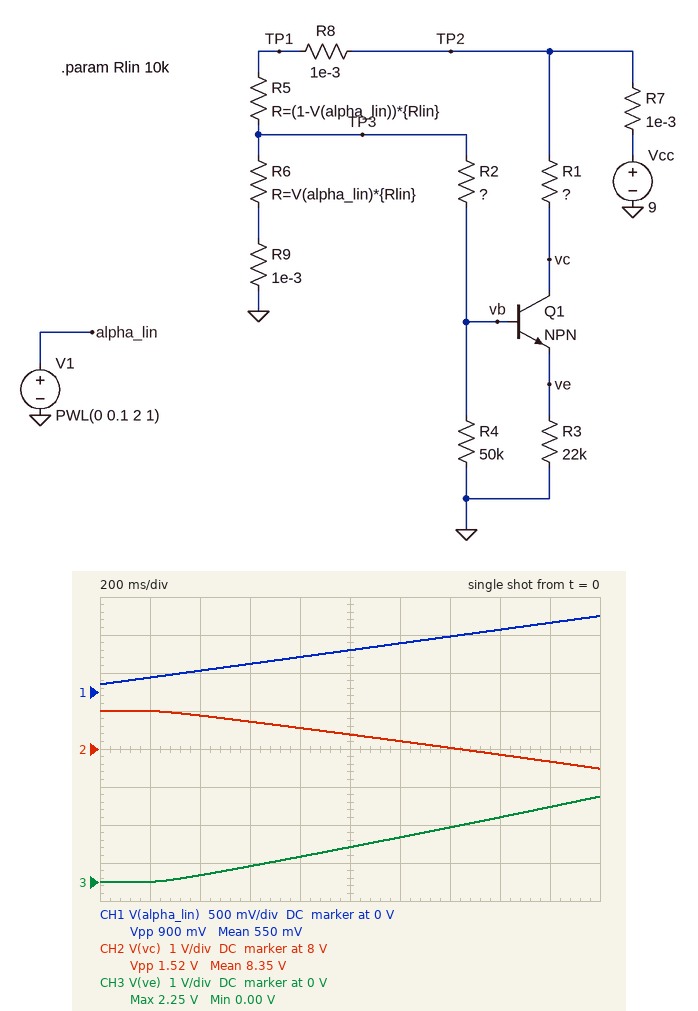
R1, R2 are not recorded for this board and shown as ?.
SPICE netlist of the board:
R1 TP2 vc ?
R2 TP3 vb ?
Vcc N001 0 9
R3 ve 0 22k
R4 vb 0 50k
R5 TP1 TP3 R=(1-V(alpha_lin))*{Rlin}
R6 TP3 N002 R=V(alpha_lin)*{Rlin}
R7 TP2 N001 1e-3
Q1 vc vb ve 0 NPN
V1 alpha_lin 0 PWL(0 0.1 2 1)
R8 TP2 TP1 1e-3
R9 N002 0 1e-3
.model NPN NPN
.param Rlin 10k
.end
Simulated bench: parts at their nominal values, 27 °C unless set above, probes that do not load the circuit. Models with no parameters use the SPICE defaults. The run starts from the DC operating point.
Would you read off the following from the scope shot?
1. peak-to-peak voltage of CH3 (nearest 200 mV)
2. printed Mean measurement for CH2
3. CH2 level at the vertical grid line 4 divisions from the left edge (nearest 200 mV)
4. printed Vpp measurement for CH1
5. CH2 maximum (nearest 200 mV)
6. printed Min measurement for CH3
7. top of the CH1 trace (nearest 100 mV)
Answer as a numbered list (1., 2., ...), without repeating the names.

1. 2.2 V
2. 8.35 V
3. 8.6 V
4. 900 mV
5. 9.0 V
6. 0.00 V
7. 1.0 V
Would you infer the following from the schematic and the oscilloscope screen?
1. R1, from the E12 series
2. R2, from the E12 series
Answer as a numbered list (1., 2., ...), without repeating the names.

1. 15 kΩ
2. 100 kΩ
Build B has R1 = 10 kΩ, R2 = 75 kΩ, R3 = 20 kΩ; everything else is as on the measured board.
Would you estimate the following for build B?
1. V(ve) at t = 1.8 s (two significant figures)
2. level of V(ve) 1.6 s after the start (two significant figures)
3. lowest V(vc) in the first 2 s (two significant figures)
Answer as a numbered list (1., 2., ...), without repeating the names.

1. 2.5 V
2. 2.2 V
3. 7.6 V
